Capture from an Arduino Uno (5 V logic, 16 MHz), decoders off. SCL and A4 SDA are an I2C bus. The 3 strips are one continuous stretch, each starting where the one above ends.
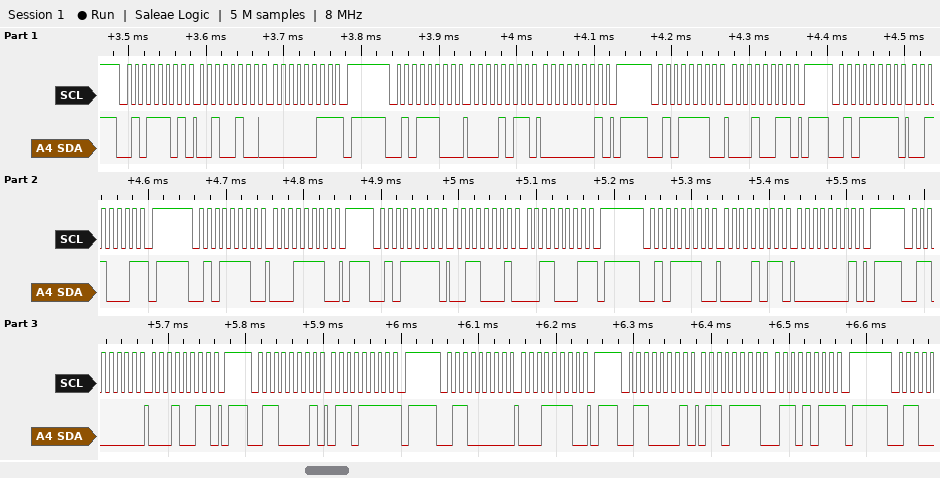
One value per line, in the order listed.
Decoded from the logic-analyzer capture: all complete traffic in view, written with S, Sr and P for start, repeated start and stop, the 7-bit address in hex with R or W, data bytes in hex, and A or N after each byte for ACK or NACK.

S 2ER A 24 A 03 N P S 2EW A 0B A 01 A P S 2FW A 13 A P S 2FR A 31 N P S 2FW A 1E A P S 2FR A 31 A 31 N P S 2FW A 0B A 01 A P S 30W A 13 A P S 30R A 6F N P S 30W A 1E A P S 30R A 6F A 6B N P
